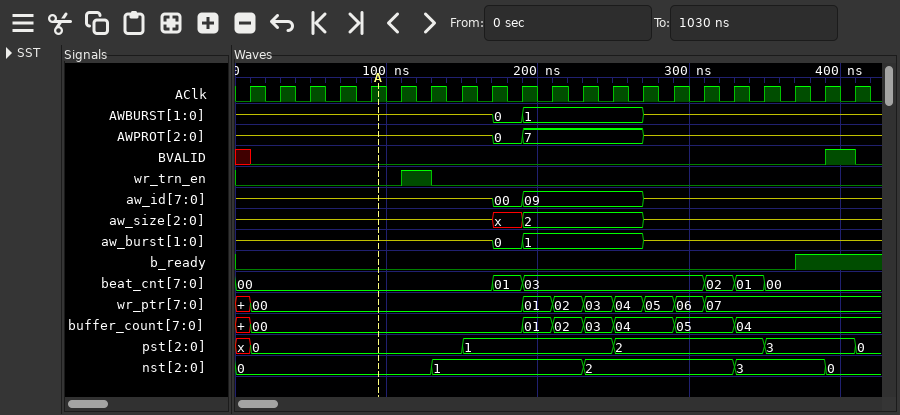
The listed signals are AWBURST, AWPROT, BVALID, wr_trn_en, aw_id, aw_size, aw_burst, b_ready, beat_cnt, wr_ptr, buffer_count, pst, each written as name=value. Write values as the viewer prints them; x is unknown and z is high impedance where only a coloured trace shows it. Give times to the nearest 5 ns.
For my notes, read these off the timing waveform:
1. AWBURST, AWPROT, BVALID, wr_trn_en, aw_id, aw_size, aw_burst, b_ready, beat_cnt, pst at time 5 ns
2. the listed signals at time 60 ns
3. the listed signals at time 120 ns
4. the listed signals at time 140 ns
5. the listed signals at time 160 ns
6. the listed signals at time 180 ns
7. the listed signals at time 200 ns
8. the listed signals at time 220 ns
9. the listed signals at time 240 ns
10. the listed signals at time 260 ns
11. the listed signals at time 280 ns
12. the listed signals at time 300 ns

AWBURST=z, AWPROT=z, BVALID=x, wr_trn_en=0, aw_id=z, aw_size=z, aw_burst=z, b_ready=0, beat_cnt=00, pst=x
AWBURST=z, AWPROT=z, BVALID=0, wr_trn_en=0, aw_id=z, aw_size=z, aw_burst=z, b_ready=0, beat_cnt=00, wr_ptr=00, buffer_count=00, pst=0
AWBURST=z, AWPROT=z, BVALID=0, wr_trn_en=1, aw_id=z, aw_size=z, aw_burst=z, b_ready=0, beat_cnt=00, wr_ptr=00, buffer_count=00, pst=0
AWBURST=z, AWPROT=z, BVALID=0, wr_trn_en=0, aw_id=z, aw_size=z, aw_burst=z, b_ready=0, beat_cnt=00, wr_ptr=00, buffer_count=00, pst=0
AWBURST=z, AWPROT=z, BVALID=0, wr_trn_en=0, aw_id=z, aw_size=z, aw_burst=z, b_ready=0, beat_cnt=00, wr_ptr=00, buffer_count=00, pst=1
AWBURST=0, AWPROT=0, BVALID=0, wr_trn_en=0, aw_id=00, aw_size=x, aw_burst=0, b_ready=0, beat_cnt=01, wr_ptr=00, buffer_count=00, pst=1
AWBURST=1, AWPROT=7, BVALID=0, wr_trn_en=0, aw_id=09, aw_size=2, aw_burst=1, b_ready=0, beat_cnt=03, wr_ptr=01, buffer_count=01, pst=1
AWBURST=1, AWPROT=7, BVALID=0, wr_trn_en=0, aw_id=09, aw_size=2, aw_burst=1, b_ready=0, beat_cnt=03, wr_ptr=02, buffer_count=02, pst=1
AWBURST=1, AWPROT=7, BVALID=0, wr_trn_en=0, aw_id=09, aw_size=2, aw_burst=1, b_ready=0, beat_cnt=03, wr_ptr=03, buffer_count=03, pst=1
AWBURST=1, AWPROT=7, BVALID=0, wr_trn_en=0, aw_id=09, aw_size=2, aw_burst=1, b_ready=0, beat_cnt=03, wr_ptr=04, buffer_count=04, pst=2
AWBURST=z, AWPROT=z, BVALID=0, wr_trn_en=0, aw_id=z, aw_size=z, aw_burst=z, b_ready=0, beat_cnt=03, wr_ptr=05, buffer_count=04, pst=2
AWBURST=z, AWPROT=z, BVALID=0, wr_trn_en=0, aw_id=z, aw_size=z, aw_burst=z, b_ready=0, beat_cnt=03, wr_ptr=06, buffer_count=05, pst=2
